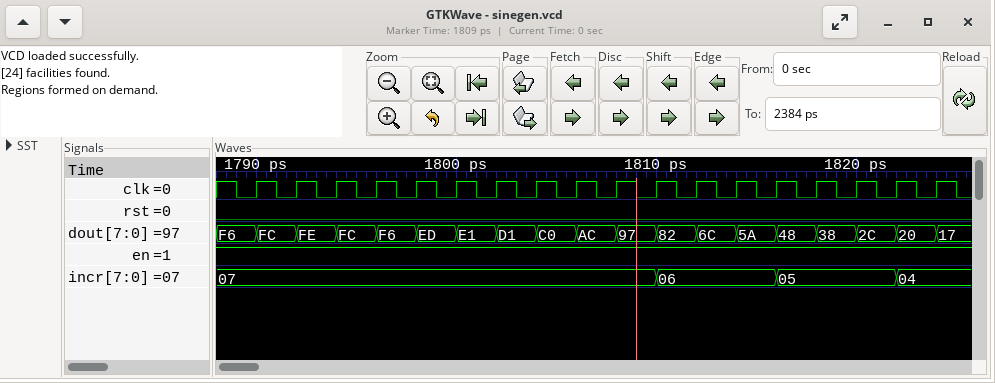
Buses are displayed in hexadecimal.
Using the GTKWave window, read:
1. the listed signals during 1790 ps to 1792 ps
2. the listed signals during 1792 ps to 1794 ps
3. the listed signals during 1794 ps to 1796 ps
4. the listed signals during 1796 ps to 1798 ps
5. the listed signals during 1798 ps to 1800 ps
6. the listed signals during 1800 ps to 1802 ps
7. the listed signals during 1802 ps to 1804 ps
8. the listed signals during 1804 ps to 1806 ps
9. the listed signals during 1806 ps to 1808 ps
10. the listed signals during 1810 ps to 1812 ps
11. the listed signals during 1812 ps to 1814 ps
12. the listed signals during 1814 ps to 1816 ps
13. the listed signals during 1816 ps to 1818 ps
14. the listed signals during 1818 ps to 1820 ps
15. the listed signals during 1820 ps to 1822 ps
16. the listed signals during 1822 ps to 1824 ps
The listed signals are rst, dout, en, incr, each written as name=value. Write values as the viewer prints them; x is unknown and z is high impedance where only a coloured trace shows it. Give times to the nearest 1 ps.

rst=0, dout=FC, en=1, incr=07
rst=0, dout=FE, en=1, incr=07
rst=0, dout=FC, en=1, incr=07
rst=0, dout=F6, en=1, incr=07
rst=0, dout=ED, en=1, incr=07
rst=0, dout=E1, en=1, incr=07
rst=0, dout=D1, en=1, incr=07
rst=0, dout=C0, en=1, incr=07
rst=0, dout=AC, en=1, incr=07
rst=0, dout=82, en=1, incr=06
rst=0, dout=6C, en=1, incr=06
rst=0, dout=5A, en=1, incr=06
rst=0, dout=48, en=1, incr=05
rst=0, dout=38, en=1, incr=05
rst=0, dout=2C, en=1, incr=05
rst=0, dout=20, en=1, incr=04
